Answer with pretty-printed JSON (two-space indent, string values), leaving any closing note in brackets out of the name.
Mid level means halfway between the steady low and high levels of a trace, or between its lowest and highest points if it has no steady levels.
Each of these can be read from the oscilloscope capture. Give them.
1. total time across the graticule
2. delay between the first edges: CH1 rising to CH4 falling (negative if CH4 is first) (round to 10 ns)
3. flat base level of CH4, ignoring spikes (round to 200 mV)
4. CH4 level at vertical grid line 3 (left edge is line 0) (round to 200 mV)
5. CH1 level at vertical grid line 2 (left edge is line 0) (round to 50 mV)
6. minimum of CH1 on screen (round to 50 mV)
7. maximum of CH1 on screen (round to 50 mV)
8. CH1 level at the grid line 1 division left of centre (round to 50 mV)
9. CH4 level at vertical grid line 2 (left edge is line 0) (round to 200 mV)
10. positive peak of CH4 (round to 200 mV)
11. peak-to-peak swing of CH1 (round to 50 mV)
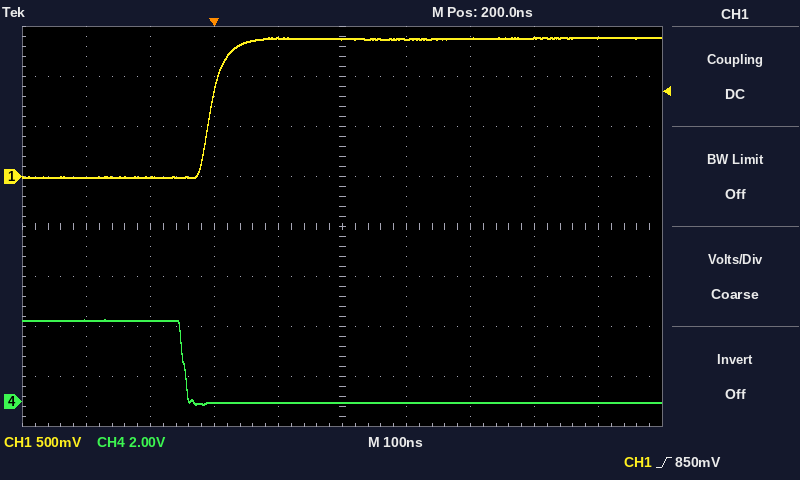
{
  "total time across the graticule": "1 µs",
  "delay between the first edges: CH1 rising to CH4 falling (negative if CH4 is first)": "-40 ns",
  "flat base level of CH4, ignoring spikes": "0.0 V",
  "CH4 level at vertical grid line 3 (left edge is line 0)": "0.0 V",
  "CH1 level at vertical grid line 2 (left edge is line 0)": "0 mV",
  "minimum of CH1 on screen": "0 mV",
  "maximum of CH1 on screen": "1.40 V",
  "CH1 level at the grid line 1 division left of centre": "1.40 V",
  "CH4 level at vertical grid line 2 (left edge is line 0)": "3.2 V",
  "positive peak of CH4": "3.2 V",
  "peak-to-peak swing of CH1": "1.40 V"
}
